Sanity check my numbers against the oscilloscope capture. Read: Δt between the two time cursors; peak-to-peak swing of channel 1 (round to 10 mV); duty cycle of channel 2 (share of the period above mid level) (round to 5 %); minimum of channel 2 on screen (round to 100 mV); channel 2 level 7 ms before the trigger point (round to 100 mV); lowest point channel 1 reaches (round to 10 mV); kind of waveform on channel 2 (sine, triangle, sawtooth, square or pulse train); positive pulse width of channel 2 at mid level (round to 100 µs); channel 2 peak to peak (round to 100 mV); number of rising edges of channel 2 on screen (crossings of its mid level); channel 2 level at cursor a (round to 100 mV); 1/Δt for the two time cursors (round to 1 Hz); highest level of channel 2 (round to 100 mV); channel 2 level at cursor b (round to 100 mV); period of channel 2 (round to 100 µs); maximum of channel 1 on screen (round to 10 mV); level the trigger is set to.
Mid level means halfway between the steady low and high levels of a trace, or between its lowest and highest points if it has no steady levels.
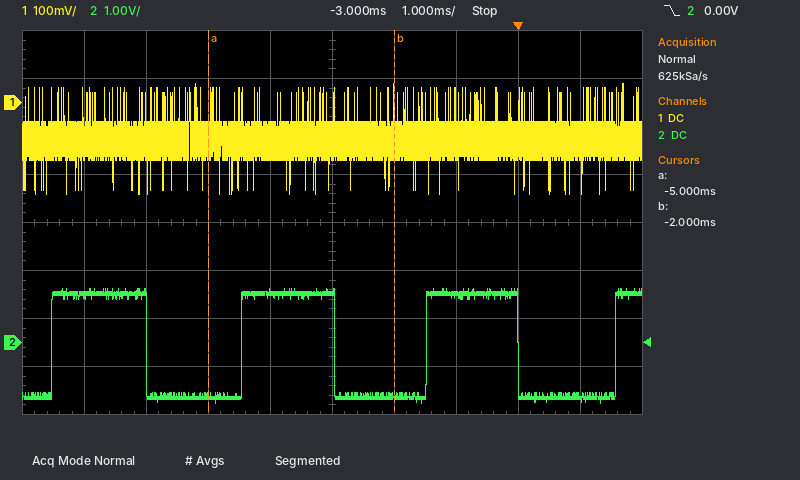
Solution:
3.0 ms
230 mV
50 %
-1.3 V
1.0 V
-190 mV
square
1.5 ms
2.4 V
4
-1.1 V
333 Hz
1.1 V
-1.1 V
3.0 ms
40 mV
0.00 V
